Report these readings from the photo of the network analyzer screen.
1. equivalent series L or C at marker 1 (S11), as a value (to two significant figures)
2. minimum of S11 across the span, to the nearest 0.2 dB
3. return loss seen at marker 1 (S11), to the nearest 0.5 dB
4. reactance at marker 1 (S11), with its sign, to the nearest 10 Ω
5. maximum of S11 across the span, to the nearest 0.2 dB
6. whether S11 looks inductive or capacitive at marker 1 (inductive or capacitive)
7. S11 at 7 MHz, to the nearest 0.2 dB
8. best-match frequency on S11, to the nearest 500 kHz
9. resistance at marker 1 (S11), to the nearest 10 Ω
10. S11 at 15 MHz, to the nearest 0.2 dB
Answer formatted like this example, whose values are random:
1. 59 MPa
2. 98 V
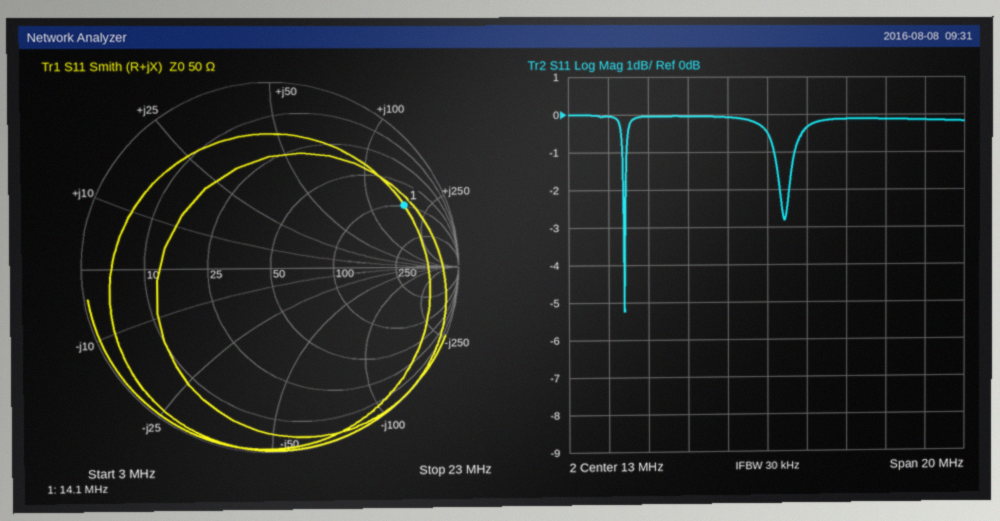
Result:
1. 1.9 µH
2. -5.2 dB
3. 2.0 dB
4. +170 Ω
5. 0.0 dB
6. inductive
7. 0.0 dB
8. 6.0 MHz
9. 100 Ω
10. -0.4 dB
